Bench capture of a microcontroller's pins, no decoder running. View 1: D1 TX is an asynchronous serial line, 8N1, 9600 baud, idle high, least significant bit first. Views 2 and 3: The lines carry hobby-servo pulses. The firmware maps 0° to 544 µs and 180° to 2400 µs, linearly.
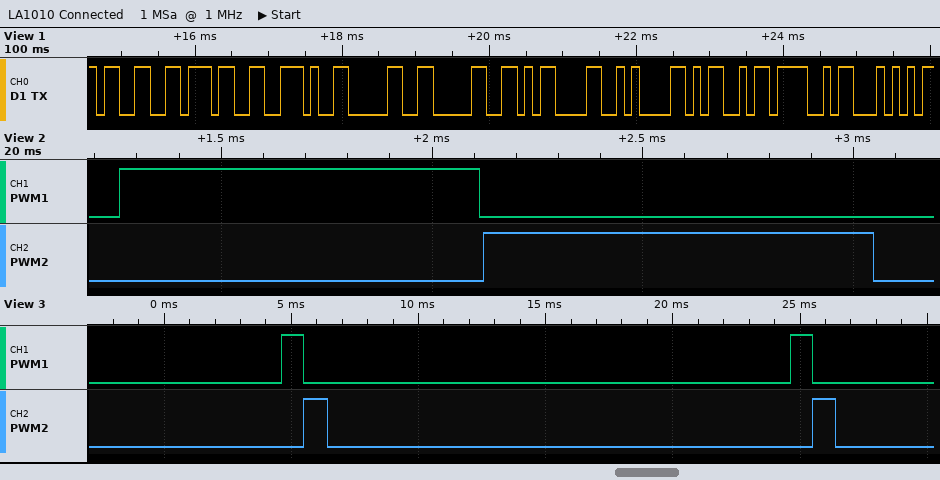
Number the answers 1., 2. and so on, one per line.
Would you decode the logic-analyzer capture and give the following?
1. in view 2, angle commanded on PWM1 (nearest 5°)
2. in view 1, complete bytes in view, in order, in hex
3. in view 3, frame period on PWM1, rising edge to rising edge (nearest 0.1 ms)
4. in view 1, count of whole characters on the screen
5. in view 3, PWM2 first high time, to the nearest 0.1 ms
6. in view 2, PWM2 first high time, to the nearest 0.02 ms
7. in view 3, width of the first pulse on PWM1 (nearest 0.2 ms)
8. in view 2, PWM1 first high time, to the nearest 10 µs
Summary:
1. 30°
2. 33 37 2E 30 30 0D 0A 4D 4F 54
3. 20.0 ms
4. 10
5. 0.9 ms
6. 0.92 ms
7. 0.8 ms
8. 850 µs
